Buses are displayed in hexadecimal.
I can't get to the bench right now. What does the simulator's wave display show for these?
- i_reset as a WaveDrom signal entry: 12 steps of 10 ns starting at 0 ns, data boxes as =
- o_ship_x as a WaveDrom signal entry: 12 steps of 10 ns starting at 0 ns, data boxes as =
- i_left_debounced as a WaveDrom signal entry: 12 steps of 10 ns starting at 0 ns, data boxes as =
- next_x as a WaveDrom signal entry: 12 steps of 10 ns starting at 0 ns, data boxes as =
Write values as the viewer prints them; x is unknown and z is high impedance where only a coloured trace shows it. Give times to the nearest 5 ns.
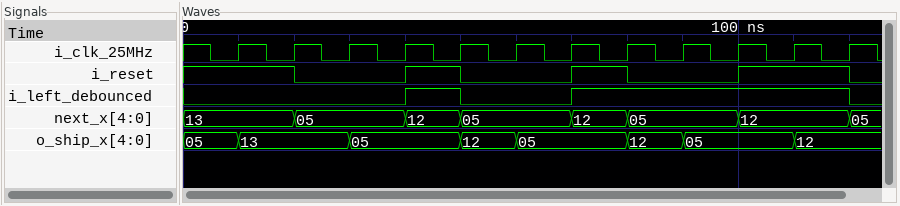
{name: 'i_reset', wave: '1.0.10.10.1.'}
{name: 'o_ship_x', wave: '==.=.==.==.=', data: '05 13 05 12 05 12 05 12'}
{name: 'i_left_debounced', wave: '0...10.1....'}
{name: 'next_x', wave: '=.=.==.==.=.', data: '13 05 12 05 12 05 12'}
